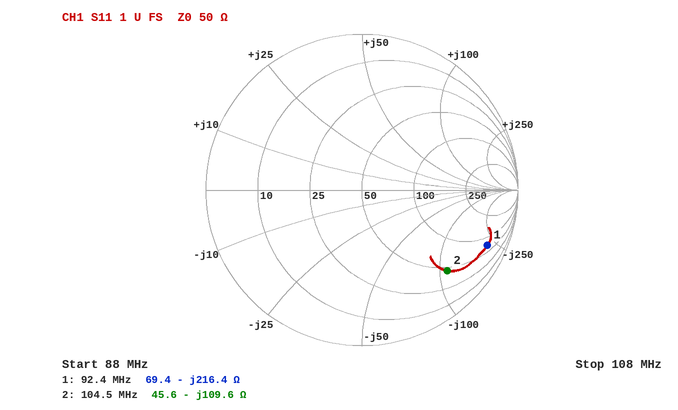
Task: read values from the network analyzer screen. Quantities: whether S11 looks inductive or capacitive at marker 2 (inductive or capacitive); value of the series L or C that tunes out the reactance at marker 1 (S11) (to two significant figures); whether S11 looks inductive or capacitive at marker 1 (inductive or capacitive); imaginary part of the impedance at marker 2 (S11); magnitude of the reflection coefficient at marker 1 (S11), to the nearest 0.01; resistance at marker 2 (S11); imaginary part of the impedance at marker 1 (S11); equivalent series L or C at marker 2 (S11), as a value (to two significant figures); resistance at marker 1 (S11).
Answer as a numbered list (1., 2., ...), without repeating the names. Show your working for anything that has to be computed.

1. capacitive
2. L = 216.4 Ω/(2π × 92.4 MHz) ≈ 373 nH, so 370 nH to two significant figures
3. capacitive
4. -109.6 Ω
5. 0.88
6. 45.6 Ω
7. -216.4 Ω
8. C = 1/(2π × 104.5 MHz × 109.6 Ω) ≈ 14 pF
9. 69.4 Ω
